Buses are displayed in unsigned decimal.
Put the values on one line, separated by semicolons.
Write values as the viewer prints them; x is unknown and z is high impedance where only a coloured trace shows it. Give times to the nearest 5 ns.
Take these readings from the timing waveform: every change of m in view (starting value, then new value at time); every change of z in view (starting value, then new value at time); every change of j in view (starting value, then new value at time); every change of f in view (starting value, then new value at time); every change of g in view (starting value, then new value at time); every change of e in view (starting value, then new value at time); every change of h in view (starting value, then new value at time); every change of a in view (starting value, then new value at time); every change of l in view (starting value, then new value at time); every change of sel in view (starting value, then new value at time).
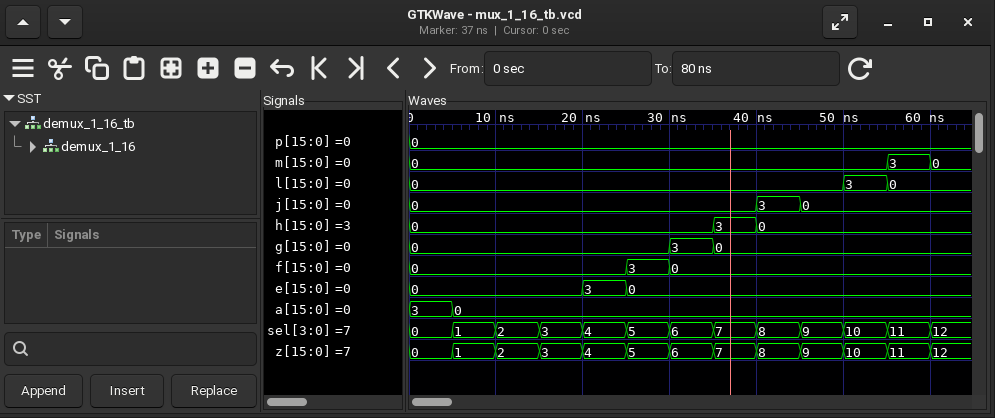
0, 3 at 55 ns, 0 at 60 ns; 0, 1 at 5 ns, 2 at 10 ns, 3 at 15 ns, 4 at 20 ns, 5 at 25 ns, 6 at 30 ns, 7 at 35 ns, 8 at 40 ns, 9 at 45 ns, 10 at 50 ns, 11 at 55 ns, 12 at 60 ns; 0, 3 at 40 ns, 0 at 45 ns; 0, 3 at 25 ns, 0 at 30 ns; 0, 3 at 30 ns, 0 at 35 ns; 0, 3 at 20 ns, 0 at 25 ns; 0, 3 at 35 ns, 0 at 40 ns; 3, 0 at 5 ns; 0, 3 at 50 ns, 0 at 55 ns; 0, 1 at 5 ns, 2 at 10 ns, 3 at 15 ns, 4 at 20 ns, 5 at 25 ns, 6 at 30 ns, 7 at 35 ns, 8 at 40 ns, 9 at 45 ns, 10 at 50 ns, 11 at 55 ns, 12 at 60 ns
